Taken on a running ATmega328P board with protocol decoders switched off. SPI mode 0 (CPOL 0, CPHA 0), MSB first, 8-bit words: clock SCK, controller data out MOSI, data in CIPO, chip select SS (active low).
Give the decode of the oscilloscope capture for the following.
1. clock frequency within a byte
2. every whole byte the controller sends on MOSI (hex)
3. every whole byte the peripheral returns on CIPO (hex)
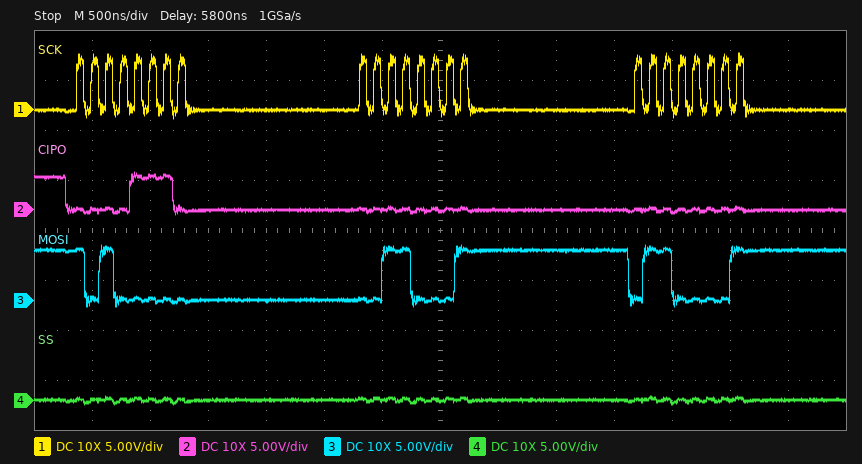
8 MHz
A0 31 61
0E 00 00
